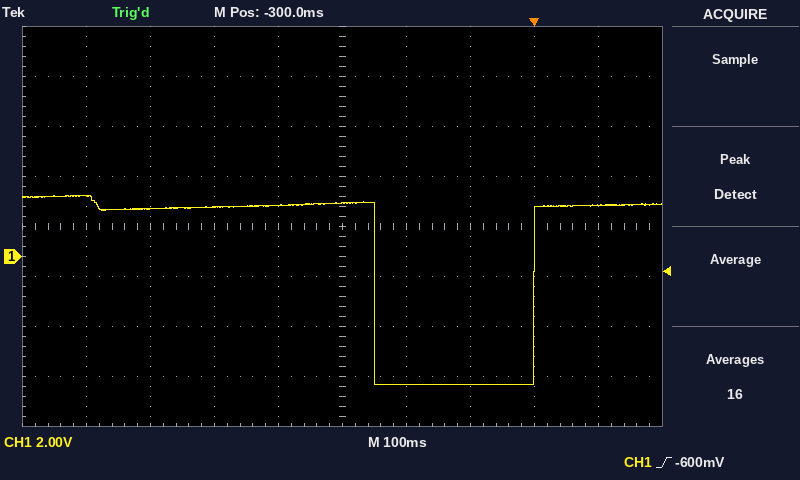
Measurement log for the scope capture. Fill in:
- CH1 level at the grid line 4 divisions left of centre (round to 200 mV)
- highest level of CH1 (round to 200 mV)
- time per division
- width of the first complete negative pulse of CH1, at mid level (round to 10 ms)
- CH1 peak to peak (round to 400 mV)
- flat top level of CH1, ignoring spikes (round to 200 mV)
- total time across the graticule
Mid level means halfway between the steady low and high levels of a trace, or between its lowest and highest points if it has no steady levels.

2.4 V
2.4 V
100 ms
250 ms
7.6 V
2.0 V
1 s
